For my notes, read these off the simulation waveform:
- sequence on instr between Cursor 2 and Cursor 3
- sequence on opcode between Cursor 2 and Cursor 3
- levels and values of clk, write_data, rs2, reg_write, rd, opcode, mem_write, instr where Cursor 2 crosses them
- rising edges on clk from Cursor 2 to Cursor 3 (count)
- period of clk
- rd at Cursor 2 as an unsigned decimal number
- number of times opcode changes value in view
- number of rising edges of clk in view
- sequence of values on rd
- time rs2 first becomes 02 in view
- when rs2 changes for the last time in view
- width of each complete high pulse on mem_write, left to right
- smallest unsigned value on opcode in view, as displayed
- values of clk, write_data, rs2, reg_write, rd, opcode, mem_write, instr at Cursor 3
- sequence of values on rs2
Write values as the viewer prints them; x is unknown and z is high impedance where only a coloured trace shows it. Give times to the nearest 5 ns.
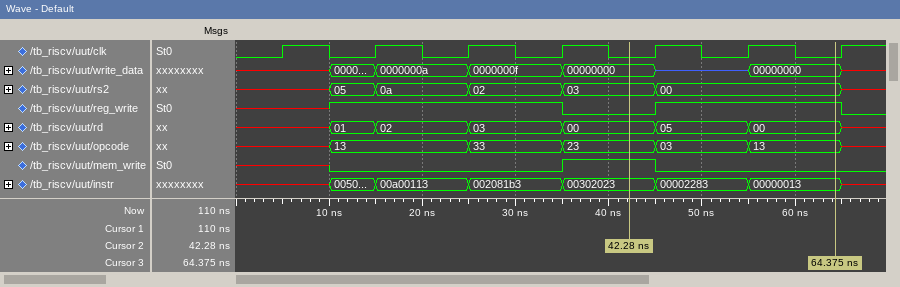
00302023, 00002283, 00000013
23, 03, 13
clk=0, write_data=00000000, rs2=03, reg_write=0, rd=00, opcode=23, mem_write=1, instr=00302023
2
10 ns
0
6
7
x, 01, 02, 03, 00, 05, 00, x
25 ns
65 ns
10 ns
03
clk=0, write_data=00000000, rs2=00, reg_write=1, rd=00, opcode=13, mem_write=0, instr=00000013
x, 05, 0a, 02, 03, 00, x
